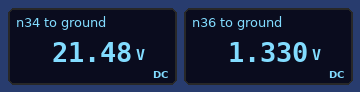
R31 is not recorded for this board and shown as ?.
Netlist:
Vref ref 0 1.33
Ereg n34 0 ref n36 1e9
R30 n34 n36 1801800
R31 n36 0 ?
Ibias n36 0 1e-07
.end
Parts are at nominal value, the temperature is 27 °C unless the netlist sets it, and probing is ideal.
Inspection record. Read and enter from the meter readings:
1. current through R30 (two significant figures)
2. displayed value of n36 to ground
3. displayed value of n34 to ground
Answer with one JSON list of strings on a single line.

["11 µA", "1.330 V", "21.48 V"]
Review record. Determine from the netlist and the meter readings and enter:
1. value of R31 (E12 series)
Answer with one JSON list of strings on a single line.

["120 kΩ"]
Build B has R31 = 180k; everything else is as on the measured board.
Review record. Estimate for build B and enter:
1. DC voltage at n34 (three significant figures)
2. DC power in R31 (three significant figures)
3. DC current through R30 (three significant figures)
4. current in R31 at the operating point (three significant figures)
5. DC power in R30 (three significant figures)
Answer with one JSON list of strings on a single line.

["14.8 V", "9.83 µW", "7.49 µA", "7.39 µA", "101 µW"]
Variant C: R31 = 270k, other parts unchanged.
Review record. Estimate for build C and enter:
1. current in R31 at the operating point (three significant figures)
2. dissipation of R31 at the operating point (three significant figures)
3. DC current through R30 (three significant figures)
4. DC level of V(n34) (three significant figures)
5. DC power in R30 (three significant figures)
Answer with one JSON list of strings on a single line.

["4.93 µA", "6.55 µW", "5.03 µA", "10.4 V", "45.5 µW"]
